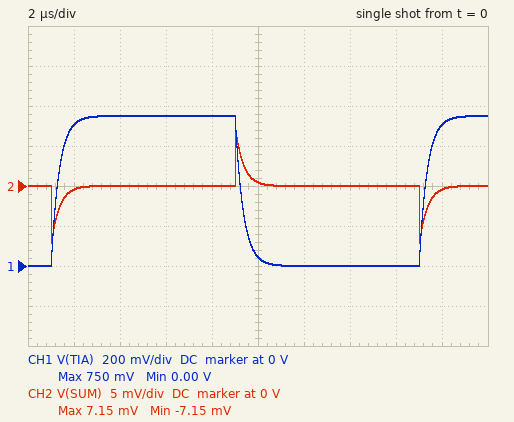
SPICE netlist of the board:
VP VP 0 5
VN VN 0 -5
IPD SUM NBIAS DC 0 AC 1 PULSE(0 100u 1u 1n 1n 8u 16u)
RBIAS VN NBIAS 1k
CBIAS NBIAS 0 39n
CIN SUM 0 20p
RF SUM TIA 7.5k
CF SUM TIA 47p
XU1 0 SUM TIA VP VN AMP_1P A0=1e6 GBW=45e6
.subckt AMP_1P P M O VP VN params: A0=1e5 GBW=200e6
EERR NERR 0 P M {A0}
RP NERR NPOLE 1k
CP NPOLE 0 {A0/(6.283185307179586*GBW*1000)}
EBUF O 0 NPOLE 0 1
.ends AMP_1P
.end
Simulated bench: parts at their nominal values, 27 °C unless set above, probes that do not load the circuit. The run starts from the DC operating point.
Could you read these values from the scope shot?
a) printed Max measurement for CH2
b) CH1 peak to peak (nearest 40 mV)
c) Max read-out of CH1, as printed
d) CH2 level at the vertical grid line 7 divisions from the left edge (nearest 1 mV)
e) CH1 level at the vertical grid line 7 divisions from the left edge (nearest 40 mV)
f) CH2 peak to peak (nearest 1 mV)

7.15 mV
760 mV
750 mV
0 V
0 V
14 mV
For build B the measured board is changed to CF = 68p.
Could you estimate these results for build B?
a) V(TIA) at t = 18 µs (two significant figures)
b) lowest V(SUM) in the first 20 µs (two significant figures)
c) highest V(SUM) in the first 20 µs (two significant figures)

640 mV
-5.0 mV
5.0 mV
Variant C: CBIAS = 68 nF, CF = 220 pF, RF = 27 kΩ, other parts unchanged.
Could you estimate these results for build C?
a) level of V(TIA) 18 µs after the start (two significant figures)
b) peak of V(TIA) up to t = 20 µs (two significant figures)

860 mV
2.0 V
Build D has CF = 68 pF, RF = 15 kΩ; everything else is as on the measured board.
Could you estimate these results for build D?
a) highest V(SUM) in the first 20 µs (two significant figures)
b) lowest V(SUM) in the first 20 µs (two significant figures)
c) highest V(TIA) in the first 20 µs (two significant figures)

5.1 mV
-5.1 mV
1.5 V
